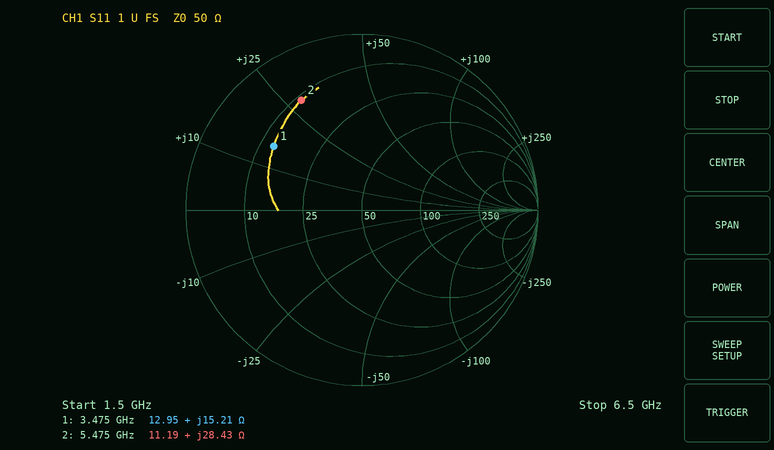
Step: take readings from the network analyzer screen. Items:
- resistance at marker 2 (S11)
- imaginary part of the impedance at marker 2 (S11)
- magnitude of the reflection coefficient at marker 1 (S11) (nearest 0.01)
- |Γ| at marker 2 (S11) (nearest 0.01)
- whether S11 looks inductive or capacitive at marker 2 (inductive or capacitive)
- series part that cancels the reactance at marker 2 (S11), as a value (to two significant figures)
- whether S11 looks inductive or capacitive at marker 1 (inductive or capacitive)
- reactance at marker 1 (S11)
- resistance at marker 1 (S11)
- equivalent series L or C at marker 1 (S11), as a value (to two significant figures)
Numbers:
11.19 Ω
+28.43 Ω
0.62
0.71
inductive
1.0 pF
inductive
+15.21 Ω
12.95 Ω
700 pH
